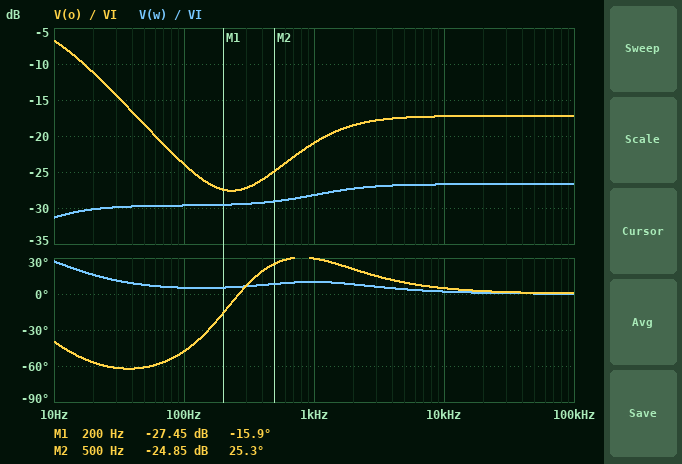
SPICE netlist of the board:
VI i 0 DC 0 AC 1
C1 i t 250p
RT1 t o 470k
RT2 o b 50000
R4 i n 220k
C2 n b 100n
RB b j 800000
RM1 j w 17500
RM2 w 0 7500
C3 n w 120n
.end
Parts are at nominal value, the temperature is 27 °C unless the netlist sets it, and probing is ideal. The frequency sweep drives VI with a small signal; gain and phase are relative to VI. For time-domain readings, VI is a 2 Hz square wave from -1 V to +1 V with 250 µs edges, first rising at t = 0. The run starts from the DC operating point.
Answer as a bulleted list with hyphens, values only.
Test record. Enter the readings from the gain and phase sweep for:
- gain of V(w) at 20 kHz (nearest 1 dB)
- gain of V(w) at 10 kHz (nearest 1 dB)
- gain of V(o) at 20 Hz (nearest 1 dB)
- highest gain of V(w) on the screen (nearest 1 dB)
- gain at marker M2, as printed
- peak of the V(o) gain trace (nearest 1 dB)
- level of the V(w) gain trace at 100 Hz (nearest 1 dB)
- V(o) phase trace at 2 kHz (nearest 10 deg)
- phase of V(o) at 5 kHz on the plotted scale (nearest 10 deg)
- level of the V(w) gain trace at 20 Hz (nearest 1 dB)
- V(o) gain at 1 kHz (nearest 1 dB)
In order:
- -27 dB
- -27 dB
- -11 dB
- -27 dB
- -24.85 dB
- -7 dB
- -30 dB
- 20 deg
- 10 deg
- -30 dB
- -21 dB
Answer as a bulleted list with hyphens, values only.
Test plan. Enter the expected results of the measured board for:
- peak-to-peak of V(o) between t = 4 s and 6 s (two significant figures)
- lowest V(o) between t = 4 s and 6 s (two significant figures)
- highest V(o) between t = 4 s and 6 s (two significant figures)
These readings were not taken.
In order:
- 1.8 V
- -910 mV
- 910 mV
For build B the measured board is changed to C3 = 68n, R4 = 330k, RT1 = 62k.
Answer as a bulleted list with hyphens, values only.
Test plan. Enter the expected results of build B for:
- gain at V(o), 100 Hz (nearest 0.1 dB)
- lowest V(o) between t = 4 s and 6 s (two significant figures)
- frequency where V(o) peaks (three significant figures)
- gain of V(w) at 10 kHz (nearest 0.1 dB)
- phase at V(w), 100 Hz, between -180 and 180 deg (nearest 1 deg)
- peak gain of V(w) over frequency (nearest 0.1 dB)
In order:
- -23.4 dB
- -870 mV
- 3.66 Hz
- -22.7 dB
- 7 deg
- -21.7 dB
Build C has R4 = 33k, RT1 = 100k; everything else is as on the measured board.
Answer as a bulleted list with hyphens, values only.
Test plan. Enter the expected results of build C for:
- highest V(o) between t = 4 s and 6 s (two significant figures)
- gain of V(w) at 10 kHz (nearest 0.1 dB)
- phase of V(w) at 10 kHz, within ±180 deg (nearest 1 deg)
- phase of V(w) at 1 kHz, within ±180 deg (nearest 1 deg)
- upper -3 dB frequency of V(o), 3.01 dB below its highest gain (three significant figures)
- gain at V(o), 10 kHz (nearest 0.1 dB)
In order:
- 1.6 V
- -13.4 dB
- 3 deg
- 4 deg
- 39.3 Hz
- -7.0 dB
